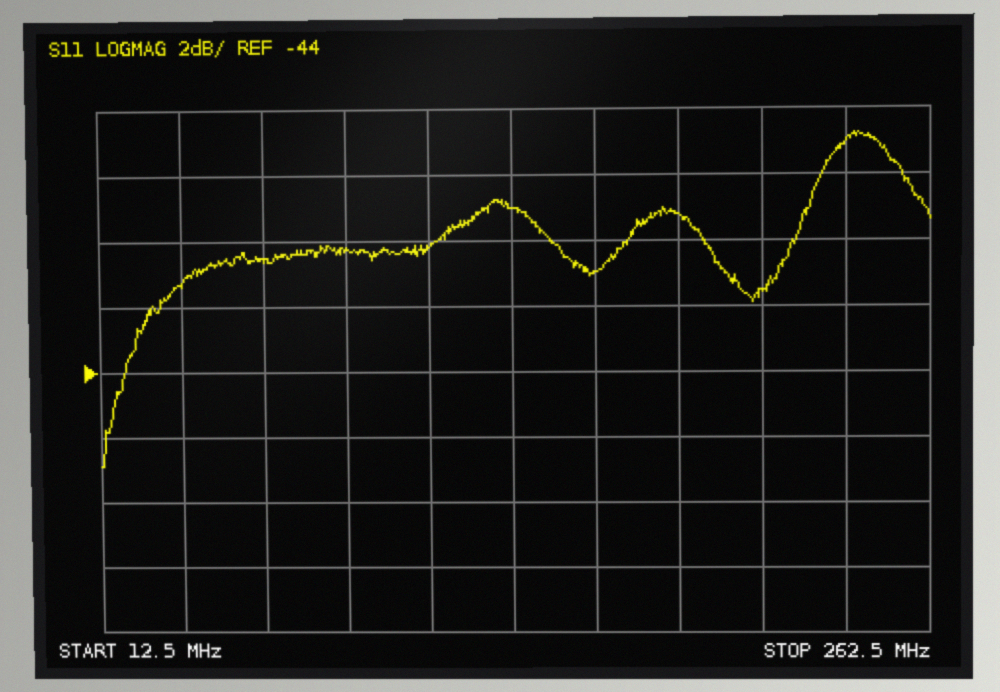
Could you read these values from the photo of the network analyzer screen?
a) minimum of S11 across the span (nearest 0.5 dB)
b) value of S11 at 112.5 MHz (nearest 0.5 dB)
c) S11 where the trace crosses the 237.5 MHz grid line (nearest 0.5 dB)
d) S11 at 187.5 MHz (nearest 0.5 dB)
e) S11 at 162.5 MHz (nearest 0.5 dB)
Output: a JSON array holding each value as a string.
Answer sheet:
["-47.0 dB", "-40.0 dB", "-37.0 dB", "-39.0 dB", "-41.0 dB"]
